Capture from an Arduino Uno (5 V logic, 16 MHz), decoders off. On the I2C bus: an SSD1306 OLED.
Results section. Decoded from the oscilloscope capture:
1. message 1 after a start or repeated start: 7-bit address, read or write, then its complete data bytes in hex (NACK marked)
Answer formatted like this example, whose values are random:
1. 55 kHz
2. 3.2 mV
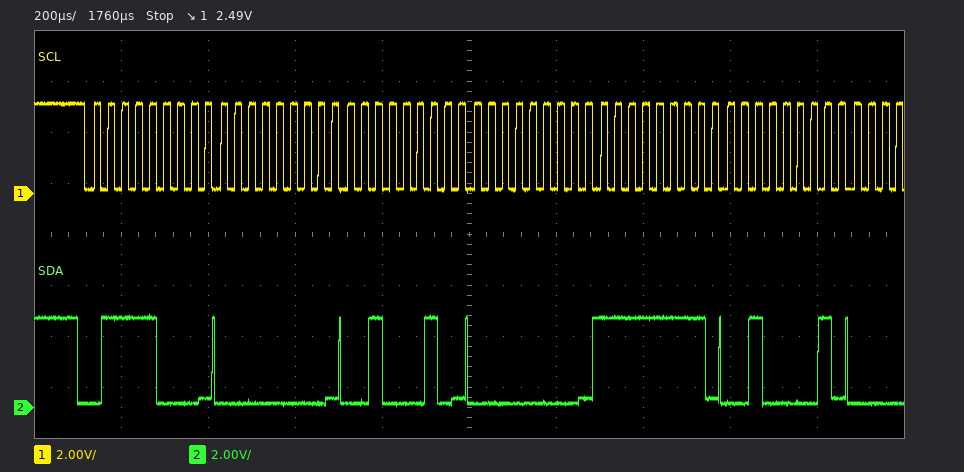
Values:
1. 0x3C write: 00 22 00 FF 21
